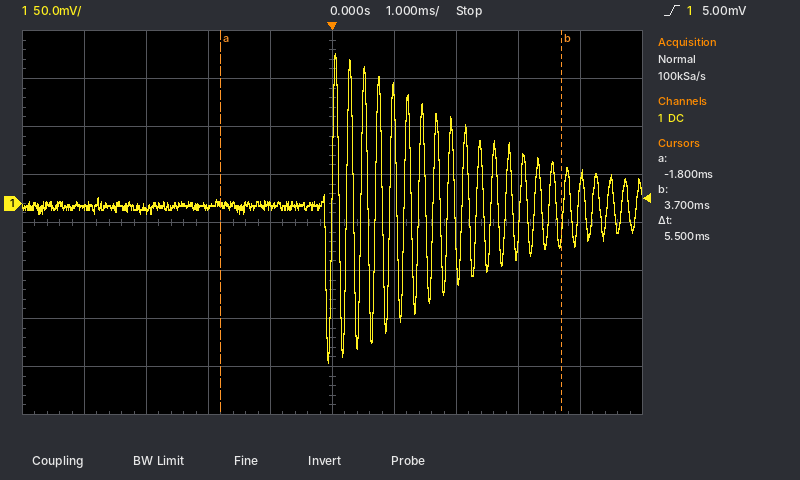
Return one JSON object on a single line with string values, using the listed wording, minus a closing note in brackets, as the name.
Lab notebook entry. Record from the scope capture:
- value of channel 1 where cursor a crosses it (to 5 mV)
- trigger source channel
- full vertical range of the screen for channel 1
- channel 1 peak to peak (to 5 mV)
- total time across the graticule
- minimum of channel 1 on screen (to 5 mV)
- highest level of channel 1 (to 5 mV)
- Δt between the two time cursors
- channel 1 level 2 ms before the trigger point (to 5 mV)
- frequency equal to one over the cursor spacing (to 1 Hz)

{"value of channel 1 where cursor a crosses it": "0 mV", "trigger source channel": "channel 1", "full vertical range of the screen for channel 1": "400 mV", "channel 1 peak to peak": "320 mV", "total time across the graticule": "10 ms", "minimum of channel 1 on screen": "-165 mV", "highest level of channel 1": "155 mV", "Δt between the two time cursors": "5.5 ms", "channel 1 level 2 ms before the trigger point": "-5 mV", "frequency equal to one over the cursor spacing": "182 Hz"}
